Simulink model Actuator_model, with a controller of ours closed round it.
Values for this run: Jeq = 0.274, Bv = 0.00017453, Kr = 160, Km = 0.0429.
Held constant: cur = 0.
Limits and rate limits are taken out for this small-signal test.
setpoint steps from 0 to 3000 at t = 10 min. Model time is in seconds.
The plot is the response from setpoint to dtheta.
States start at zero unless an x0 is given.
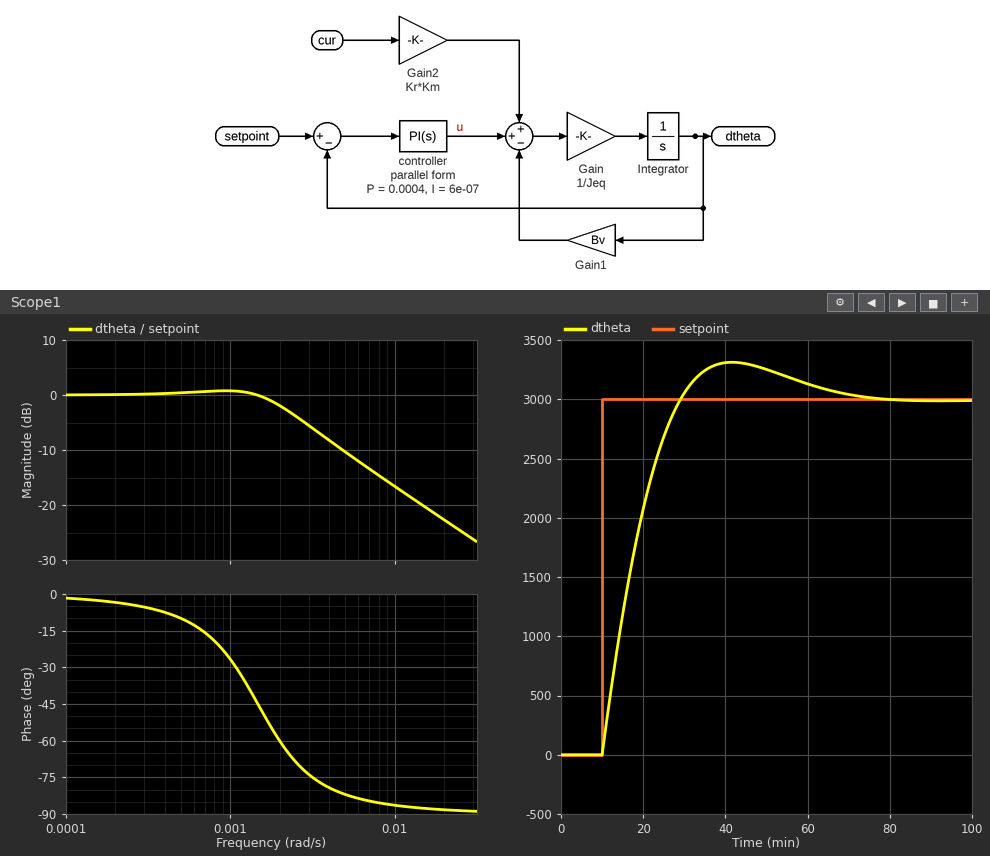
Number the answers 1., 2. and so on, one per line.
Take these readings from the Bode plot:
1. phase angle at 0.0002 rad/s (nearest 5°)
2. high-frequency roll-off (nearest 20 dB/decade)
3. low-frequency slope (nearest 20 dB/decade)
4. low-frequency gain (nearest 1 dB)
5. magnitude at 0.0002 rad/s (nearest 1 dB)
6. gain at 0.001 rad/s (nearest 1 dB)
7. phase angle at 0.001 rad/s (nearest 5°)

1. -5°
2. -20 dB/decade
3. 0 dB/decade
4. 0 dB
5. 0 dB
6. 1 dB
7. -25°
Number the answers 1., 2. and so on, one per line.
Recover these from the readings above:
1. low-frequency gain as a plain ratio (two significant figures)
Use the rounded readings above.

1. 1.0
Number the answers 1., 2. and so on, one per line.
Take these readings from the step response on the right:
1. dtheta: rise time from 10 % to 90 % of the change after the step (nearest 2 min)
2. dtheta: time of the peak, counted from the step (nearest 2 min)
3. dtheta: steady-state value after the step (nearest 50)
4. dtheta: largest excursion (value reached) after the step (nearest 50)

1. 14 min
2. 32 min
3. 3000
4. 3300
